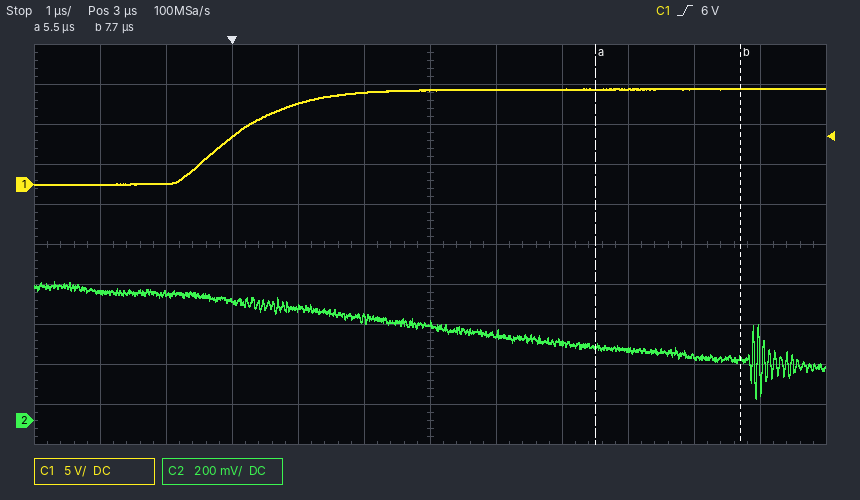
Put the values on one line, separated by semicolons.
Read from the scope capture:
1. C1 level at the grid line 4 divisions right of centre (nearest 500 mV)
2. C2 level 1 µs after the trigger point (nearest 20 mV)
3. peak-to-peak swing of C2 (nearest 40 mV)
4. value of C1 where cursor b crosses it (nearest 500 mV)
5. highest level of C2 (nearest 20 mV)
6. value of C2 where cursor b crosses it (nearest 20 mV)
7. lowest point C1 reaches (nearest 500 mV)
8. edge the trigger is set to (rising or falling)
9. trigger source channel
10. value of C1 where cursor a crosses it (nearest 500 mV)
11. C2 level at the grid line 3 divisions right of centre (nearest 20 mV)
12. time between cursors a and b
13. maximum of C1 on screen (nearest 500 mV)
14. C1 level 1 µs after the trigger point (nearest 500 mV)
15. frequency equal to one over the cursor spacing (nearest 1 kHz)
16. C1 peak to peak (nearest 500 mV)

12.0 V; 560 mV; 600 mV; 12.0 V; 700 mV; 300 mV; 0.0 V; rising; C1; 12.0 V; 360 mV; 2.2 µs; 12.0 V; 10.0 V; 455 kHz; 12.0 V
